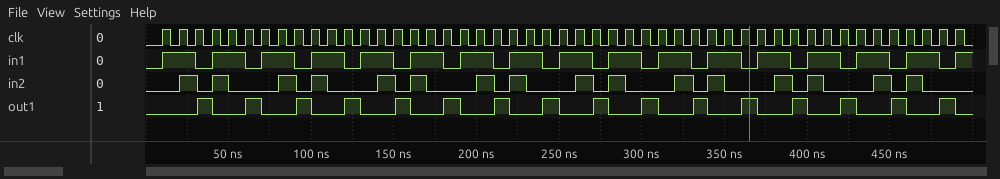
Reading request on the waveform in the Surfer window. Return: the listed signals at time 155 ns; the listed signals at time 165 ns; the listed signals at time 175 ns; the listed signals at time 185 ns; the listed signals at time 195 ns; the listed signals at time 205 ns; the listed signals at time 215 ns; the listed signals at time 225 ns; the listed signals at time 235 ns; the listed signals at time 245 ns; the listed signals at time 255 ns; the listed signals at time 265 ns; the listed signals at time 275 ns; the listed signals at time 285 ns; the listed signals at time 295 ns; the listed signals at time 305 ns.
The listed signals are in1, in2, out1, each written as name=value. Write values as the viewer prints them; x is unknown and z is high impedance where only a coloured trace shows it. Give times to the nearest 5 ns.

in1=0, in2=0, out1=1
in1=1, in2=1, out1=0
in1=1, in2=0, out1=0
in1=0, in2=0, out1=1
in1=1, in2=0, out1=0
in1=1, in2=1, out1=0
in1=0, in2=0, out1=1
in1=1, in2=1, out1=0
in1=1, in2=0, out1=0
in1=0, in2=0, out1=1
in1=1, in2=0, out1=0
in1=1, in2=1, out1=0
in1=0, in2=0, out1=1
in1=1, in2=1, out1=0
in1=1, in2=0, out1=0
in1=0, in2=0, out1=1
